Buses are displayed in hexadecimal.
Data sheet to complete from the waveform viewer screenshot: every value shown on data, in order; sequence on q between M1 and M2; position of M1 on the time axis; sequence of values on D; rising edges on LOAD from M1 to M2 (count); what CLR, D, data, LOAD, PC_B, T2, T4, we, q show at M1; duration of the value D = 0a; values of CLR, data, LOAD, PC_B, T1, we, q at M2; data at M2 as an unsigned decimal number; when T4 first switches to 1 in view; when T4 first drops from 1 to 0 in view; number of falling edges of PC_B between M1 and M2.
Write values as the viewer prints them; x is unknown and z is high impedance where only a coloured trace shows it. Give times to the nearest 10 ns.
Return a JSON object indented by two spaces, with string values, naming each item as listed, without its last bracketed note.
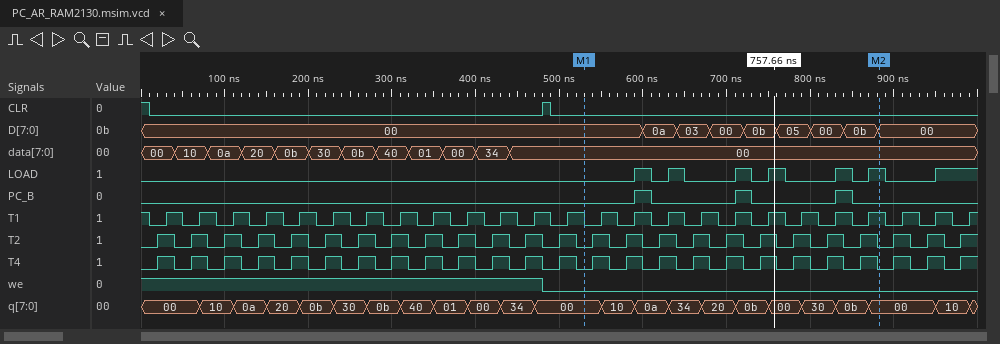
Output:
{
  "every value shown on data, in order": "00, 10, 0a, 20, 0b, 30, 0b, 40, 01, 00, 34, 00",
  "sequence on q between M1 and M2": "00, 10, 0a, 34, 20, 0b, 00, 30, 0b, 00",
  "position of M1 on the time axis": "530 ns",
  "sequence of values on D": "00, 0a, 03, 00, 0b, 05, 00, 0b, 00",
  "rising edges on LOAD from M1 to M2": "6",
  "what CLR, D, data, LOAD, PC_B, T2, T4, we, q show at M1": "CLR=0, D=00, data=00, LOAD=0, PC_B=0, T2=0, T4=0, we=0, q=00",
  "duration of the value D = 0a": "40 ns",
  "values of CLR, data, LOAD, PC_B, T1, we, q at M2": "CLR=0, data=00, LOAD=1, PC_B=0, T1=1, we=0, q=00",
  "data at M2 as an unsigned decimal number": "0",
  "when T4 first switches to 1 in view": "20 ns",
  "when T4 first drops from 1 to 0 in view": "40 ns",
  "number of falling edges of PC_B between M1 and M2": "3"
}
